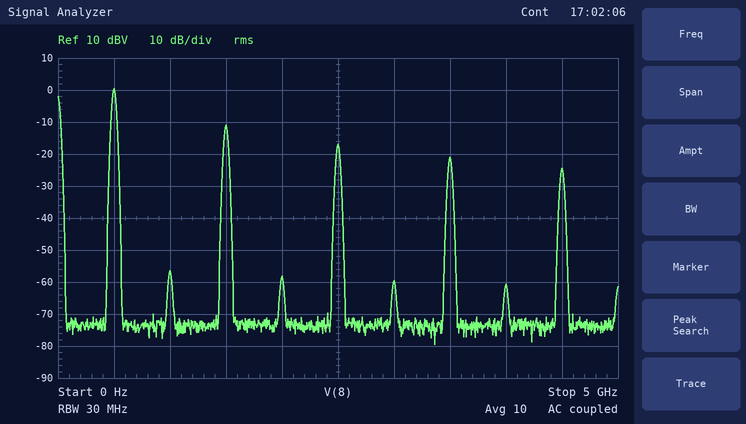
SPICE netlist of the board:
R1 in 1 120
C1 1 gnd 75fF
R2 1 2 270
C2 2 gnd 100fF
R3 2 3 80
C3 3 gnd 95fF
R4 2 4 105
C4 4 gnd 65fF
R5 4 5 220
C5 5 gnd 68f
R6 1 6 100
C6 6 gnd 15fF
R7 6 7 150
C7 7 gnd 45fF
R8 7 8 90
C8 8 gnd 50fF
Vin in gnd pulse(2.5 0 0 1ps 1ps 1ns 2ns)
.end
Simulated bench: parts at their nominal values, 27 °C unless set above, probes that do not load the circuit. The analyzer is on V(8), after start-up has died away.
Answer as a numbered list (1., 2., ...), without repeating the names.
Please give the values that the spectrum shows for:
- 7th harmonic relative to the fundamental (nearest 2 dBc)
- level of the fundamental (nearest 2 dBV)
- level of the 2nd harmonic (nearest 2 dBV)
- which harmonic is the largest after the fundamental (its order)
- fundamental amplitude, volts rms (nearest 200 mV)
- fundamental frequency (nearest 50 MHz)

1. -22 dBc
2. 0 dBV
3. -56 dBV
4. 3
5. 1.0 V
6. 500 MHz
